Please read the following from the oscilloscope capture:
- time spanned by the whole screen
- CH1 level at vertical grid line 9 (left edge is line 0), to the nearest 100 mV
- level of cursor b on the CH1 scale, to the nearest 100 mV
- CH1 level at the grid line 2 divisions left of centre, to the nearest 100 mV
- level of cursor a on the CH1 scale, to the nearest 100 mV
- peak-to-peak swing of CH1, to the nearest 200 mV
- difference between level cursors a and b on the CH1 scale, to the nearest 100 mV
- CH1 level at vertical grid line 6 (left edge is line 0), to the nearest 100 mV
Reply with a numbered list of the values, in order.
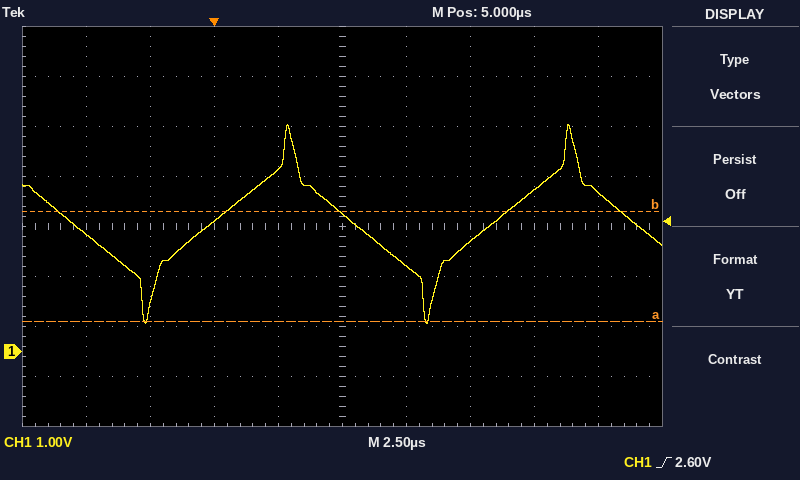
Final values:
1. 25 µs
2. 3.2 V
3. 2.8 V
4. 2.6 V
5. 600 mV
6. 4.0 V
7. 2.2 V
8. 1.7 V
